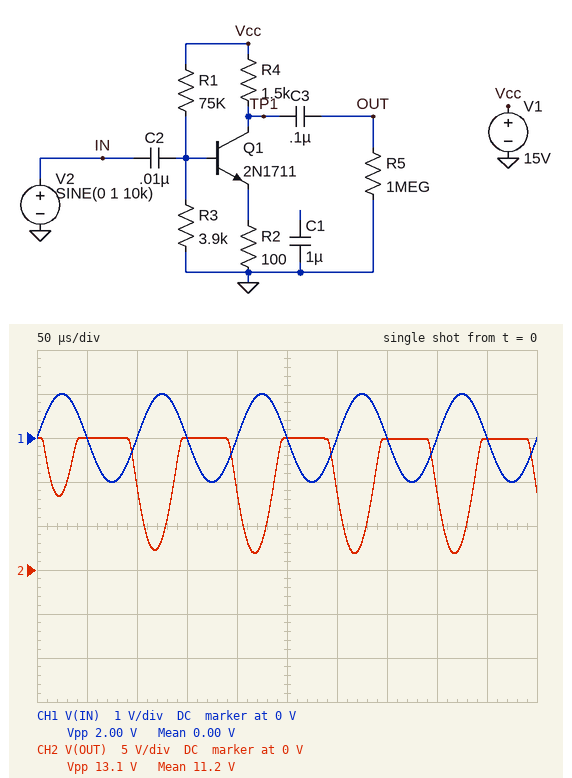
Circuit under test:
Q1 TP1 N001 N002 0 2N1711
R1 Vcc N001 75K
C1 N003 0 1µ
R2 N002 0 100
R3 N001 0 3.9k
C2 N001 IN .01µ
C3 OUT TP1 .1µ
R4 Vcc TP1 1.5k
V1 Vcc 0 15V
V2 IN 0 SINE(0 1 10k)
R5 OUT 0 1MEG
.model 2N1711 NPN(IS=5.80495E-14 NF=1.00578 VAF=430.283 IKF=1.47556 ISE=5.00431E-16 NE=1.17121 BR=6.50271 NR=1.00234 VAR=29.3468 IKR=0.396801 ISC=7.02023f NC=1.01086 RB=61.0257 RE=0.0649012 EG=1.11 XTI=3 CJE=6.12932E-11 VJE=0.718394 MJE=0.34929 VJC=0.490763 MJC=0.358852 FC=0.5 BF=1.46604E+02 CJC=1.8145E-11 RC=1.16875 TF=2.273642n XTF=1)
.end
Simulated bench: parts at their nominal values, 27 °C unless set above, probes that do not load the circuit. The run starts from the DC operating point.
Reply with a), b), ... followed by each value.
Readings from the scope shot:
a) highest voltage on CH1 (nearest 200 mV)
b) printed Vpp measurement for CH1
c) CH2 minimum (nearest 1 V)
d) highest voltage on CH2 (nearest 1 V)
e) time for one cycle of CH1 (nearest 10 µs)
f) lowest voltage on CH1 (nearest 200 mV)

a) 1.0 V
b) 2.00 V
c) 2 V
d) 15 V
e) 100 µs
f) -1.0 V
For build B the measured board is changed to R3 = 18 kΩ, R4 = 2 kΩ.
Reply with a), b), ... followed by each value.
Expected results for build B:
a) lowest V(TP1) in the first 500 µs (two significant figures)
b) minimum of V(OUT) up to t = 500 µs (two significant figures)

a) 810 mV
b) 760 mV
